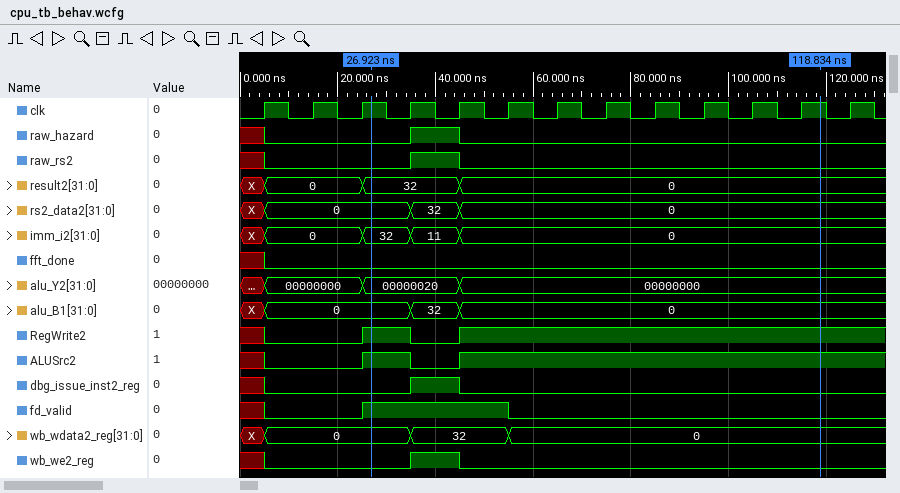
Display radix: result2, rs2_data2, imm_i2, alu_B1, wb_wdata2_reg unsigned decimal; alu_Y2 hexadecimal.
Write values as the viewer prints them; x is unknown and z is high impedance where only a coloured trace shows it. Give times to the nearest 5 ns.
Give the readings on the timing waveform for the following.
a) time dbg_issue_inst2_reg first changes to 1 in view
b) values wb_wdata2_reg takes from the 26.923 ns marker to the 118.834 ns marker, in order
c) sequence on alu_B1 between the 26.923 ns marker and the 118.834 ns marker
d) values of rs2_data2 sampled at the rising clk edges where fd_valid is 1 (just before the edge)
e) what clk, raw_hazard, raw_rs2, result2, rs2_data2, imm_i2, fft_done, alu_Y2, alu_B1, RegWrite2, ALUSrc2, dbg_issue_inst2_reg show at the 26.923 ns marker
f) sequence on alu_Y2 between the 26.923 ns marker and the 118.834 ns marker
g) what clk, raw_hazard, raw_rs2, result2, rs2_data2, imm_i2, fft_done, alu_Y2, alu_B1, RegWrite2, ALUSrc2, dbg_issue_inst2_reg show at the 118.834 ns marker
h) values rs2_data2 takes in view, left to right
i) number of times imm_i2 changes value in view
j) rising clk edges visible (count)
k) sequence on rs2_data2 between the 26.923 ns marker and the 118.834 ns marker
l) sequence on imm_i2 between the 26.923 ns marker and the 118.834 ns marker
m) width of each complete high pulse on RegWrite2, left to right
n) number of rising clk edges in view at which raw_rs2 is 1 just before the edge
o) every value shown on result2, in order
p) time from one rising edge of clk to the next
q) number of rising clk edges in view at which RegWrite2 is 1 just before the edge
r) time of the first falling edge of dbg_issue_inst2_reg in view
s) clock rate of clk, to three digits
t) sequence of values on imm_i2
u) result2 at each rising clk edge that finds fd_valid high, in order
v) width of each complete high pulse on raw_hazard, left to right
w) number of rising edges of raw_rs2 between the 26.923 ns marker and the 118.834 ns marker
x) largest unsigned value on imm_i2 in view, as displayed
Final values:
35 ns
0, 32, 0
0, 32, 0
0, 32, 0
clk=1, raw_hazard=0, raw_rs2=0, result2=32, rs2_data2=0, imm_i2=32, fft_done=0, alu_Y2=00000020, alu_B1=0, RegWrite2=1, ALUSrc2=1, dbg_issue_inst2_reg=0
00000020, 00000000
clk=1, raw_hazard=0, raw_rs2=0, result2=0, rs2_data2=0, imm_i2=0, fft_done=0, alu_Y2=00000000, alu_B1=0, RegWrite2=1, ALUSrc2=1, dbg_issue_inst2_reg=0
X, 0, 32, 0
4
13
0, 32, 0
32, 11, 0
10 ns
1
X, 0, 32, 0
10 ns
9
45 ns
100 MHz
X, 0, 32, 11, 0
32, 32, 0
10 ns
1
32
